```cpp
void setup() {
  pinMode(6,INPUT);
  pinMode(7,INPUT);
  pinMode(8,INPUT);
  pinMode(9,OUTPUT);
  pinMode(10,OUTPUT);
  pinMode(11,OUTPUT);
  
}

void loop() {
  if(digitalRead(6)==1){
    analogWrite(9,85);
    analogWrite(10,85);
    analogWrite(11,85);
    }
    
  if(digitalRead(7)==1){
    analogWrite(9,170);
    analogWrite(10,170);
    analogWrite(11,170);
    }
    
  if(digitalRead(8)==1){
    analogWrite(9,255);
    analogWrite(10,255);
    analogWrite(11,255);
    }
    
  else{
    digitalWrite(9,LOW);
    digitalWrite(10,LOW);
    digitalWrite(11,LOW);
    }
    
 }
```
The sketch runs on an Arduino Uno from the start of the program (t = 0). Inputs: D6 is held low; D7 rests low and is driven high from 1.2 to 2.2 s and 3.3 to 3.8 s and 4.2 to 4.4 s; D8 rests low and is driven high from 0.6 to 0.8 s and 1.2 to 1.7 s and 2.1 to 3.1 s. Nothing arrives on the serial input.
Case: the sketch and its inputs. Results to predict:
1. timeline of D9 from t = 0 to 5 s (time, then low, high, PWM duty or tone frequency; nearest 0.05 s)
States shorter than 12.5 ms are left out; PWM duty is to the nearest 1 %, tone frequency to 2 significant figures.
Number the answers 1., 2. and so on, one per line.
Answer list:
1. 0 s low; 0.6 s high; 0.8 s low; 2.2 s high; 3.1 s low
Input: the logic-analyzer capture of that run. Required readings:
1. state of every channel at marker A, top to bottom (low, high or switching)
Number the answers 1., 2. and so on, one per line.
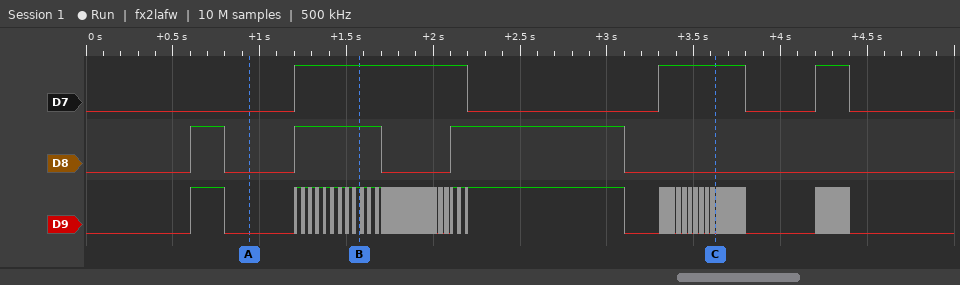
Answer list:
1. D7 low, D8 low, D9 low
